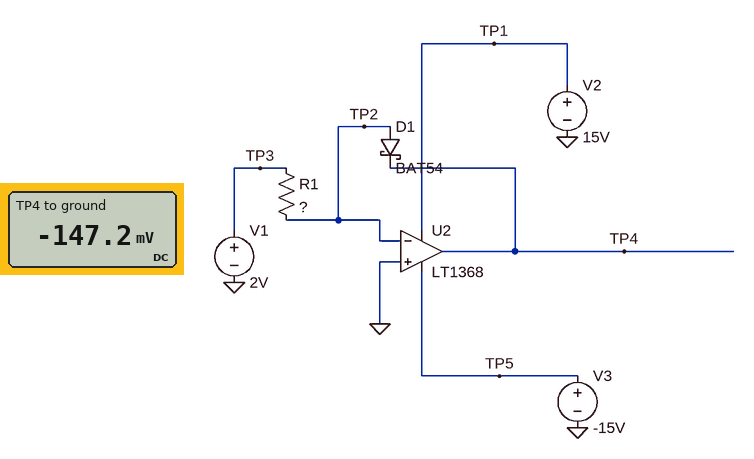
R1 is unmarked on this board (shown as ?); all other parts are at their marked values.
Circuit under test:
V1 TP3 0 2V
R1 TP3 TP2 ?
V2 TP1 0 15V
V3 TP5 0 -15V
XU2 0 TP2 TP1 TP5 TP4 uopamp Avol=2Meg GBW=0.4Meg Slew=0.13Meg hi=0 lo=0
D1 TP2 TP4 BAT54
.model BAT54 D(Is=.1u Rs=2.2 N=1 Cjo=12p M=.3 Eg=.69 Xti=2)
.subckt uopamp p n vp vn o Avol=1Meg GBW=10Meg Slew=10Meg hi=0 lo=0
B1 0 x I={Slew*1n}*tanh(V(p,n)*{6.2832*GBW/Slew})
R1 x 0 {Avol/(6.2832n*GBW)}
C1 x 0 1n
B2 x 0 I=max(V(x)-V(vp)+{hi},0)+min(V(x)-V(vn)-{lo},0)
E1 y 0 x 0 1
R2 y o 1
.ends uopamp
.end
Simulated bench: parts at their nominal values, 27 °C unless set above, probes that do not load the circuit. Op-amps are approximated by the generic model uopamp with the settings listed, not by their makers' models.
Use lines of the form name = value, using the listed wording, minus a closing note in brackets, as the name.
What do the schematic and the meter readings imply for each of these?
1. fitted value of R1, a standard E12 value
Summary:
fitted value of R1, a standard E12 value = 68 kΩ
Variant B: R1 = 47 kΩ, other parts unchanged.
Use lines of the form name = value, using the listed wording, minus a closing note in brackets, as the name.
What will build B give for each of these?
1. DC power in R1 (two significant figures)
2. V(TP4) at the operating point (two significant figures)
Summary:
DC power in R1 = 85 µW
V(TP4) at the operating point = -160 mV
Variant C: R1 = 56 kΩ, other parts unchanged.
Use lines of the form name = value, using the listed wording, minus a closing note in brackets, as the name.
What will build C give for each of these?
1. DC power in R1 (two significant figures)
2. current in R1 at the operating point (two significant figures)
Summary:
DC power in R1 = 71 µW
current in R1 at the operating point = 36 µA
